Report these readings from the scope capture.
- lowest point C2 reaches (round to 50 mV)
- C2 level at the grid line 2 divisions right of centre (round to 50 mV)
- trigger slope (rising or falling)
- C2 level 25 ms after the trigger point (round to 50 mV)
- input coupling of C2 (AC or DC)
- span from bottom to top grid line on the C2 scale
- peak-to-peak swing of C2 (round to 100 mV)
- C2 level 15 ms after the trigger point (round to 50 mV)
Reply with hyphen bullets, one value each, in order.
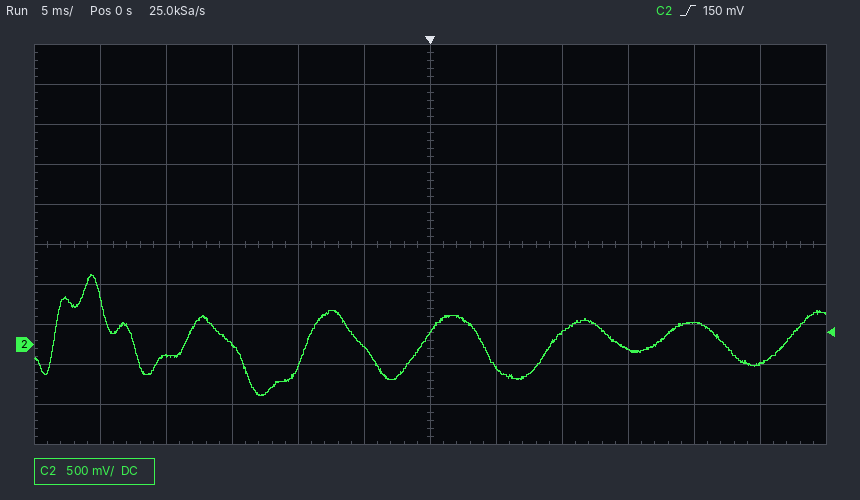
- -650 mV
- 150 mV
- rising
- -250 mV
- DC
- 5 V
- 1.50 V
- -50 mV
